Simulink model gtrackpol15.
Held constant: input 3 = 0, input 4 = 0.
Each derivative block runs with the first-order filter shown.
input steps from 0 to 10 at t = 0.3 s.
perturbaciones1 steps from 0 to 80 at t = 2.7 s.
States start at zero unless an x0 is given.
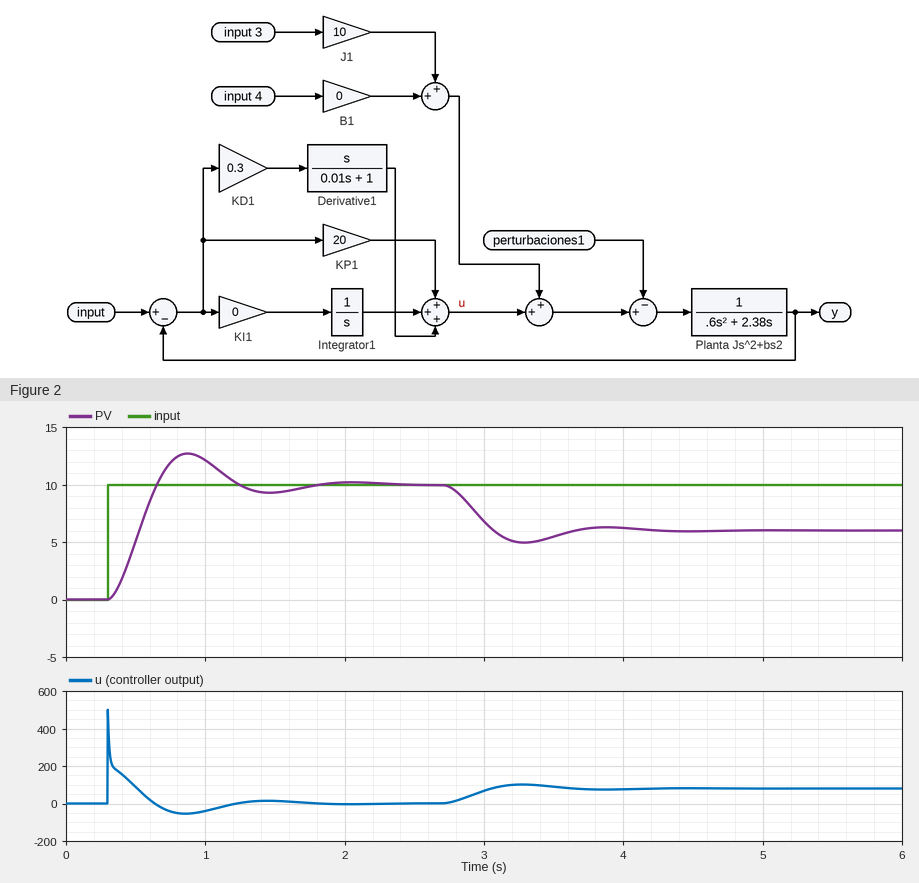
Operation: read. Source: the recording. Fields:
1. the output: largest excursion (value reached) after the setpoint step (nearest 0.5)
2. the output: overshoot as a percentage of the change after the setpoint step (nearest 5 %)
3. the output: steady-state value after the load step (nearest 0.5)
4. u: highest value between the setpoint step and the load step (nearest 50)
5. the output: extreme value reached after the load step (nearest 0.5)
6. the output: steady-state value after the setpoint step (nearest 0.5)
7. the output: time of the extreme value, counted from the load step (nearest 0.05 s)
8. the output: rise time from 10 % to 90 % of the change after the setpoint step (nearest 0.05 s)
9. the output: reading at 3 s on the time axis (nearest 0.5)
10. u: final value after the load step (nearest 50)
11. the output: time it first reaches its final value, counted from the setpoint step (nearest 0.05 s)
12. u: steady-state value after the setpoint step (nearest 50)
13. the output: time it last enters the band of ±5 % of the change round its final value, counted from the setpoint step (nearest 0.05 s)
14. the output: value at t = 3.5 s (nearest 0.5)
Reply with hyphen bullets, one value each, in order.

- 12.5
- 25 %
- 6.0
- 500
- 5.0
- 10.0
- 0.60 s
- 0.25 s
- 7.0
- 100
- 0.35 s
- 0
- 1.30 s
- 5.5
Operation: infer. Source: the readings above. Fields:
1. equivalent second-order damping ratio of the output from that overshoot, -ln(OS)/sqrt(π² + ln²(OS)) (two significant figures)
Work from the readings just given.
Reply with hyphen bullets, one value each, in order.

- 0.40
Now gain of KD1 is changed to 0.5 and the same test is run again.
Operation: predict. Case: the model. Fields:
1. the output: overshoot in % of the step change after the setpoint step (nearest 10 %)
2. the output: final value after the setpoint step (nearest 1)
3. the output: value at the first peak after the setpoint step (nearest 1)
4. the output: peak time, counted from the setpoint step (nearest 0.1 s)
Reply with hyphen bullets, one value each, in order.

- 20 %
- 10
- 12
- 0.6 s
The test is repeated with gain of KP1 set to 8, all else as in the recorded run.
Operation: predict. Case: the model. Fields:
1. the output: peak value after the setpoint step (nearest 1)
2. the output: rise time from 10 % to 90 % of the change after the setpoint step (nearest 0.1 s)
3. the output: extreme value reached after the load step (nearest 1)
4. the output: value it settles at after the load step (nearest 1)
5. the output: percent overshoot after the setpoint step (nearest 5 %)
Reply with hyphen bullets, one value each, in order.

- 11
- 0.5 s
- -1
- 0
- 10 %
